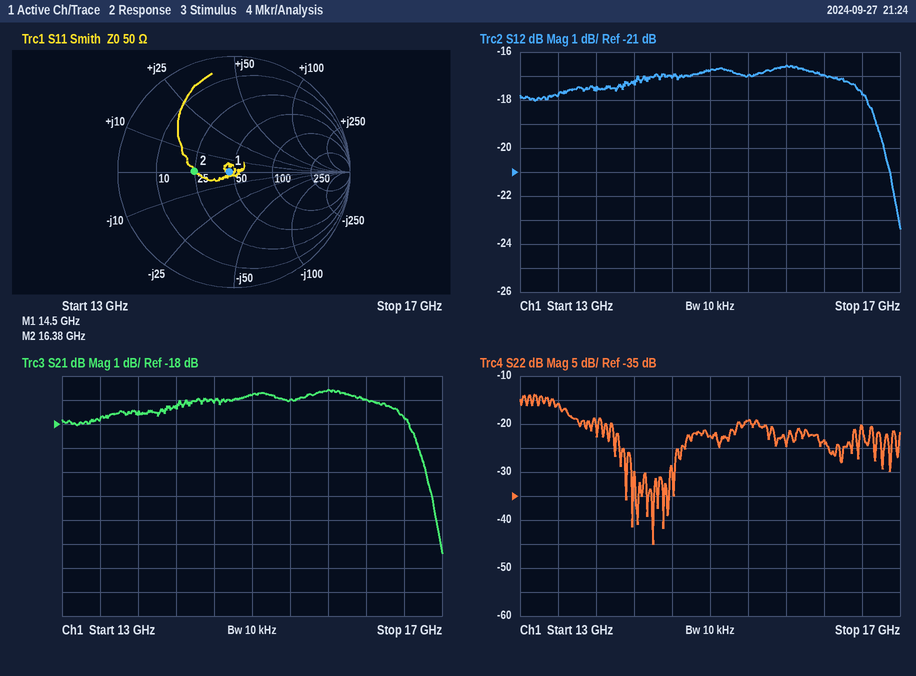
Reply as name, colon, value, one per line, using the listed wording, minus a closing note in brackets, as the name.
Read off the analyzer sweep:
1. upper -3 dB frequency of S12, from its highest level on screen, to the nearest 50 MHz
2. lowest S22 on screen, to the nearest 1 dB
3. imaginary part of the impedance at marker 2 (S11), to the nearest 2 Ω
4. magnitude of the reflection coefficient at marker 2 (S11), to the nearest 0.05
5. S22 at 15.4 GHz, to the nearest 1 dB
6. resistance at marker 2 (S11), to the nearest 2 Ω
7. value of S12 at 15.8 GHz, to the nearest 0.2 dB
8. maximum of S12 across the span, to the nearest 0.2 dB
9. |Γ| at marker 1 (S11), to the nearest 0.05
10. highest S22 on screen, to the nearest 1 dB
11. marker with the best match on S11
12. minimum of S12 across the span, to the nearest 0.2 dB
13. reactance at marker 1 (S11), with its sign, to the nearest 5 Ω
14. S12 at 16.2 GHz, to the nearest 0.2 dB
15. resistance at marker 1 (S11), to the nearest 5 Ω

upper -3 dB frequency of S12, from its highest level on screen, to the nearest 50 MHz: 16.80 GHz
lowest S22 on screen, to the nearest 1 dB: -45 dB
imaginary part of the impedance at marker 2 (S11), to the nearest 2 Ω: 0 Ω
magnitude of the reflection coefficient at marker 2 (S11), to the nearest 0.05: 0.35
S22 at 15.4 GHz, to the nearest 1 dB: -19 dB
resistance at marker 2 (S11), to the nearest 2 Ω: 24 Ω
value of S12 at 15.8 GHz, to the nearest 0.2 dB: -16.6 dB
maximum of S12 across the span, to the nearest 0.2 dB: -16.6 dB
|Γ| at marker 1 (S11), to the nearest 0.05: 0.05
highest S22 on screen, to the nearest 1 dB: -14 dB
marker with the best match on S11: marker 1
minimum of S12 across the span, to the nearest 0.2 dB: -23.4 dB
reactance at marker 1 (S11), with its sign, to the nearest 5 Ω: 0 Ω
S12 at 16.2 GHz, to the nearest 0.2 dB: -17.0 dB
resistance at marker 1 (S11), to the nearest 5 Ω: 45 Ω
